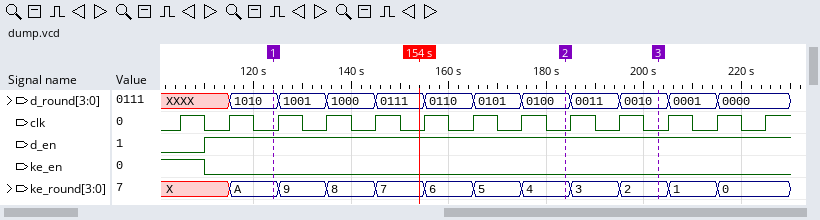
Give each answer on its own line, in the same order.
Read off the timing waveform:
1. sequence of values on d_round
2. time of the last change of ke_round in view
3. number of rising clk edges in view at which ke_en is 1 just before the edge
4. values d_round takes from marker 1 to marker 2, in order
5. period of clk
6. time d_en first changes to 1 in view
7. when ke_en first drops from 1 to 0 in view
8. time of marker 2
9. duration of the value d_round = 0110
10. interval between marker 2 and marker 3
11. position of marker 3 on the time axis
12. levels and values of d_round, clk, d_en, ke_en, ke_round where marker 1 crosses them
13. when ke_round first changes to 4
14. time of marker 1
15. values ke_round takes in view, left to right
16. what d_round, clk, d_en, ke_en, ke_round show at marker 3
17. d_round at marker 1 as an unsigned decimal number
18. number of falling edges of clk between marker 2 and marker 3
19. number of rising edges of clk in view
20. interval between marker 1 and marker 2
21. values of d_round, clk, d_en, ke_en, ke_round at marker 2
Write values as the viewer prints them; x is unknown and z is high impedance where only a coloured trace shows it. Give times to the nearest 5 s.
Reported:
XXXX, 1010, 1001, 1000, 0111, 0110, 0101, 0100, 0011, 0010, 0001, 0000
215 s
1
1010, 1001, 1000, 0111, 0110, 0101, 0100
10 s
110 s
110 s
185 s
10 s
20 s
205 s
d_round=1010, clk=0, d_en=1, ke_en=0, ke_round=A
175 s
125 s
X, A, 9, 8, 7, 6, 5, 4, 3, 2, 1, 0
d_round=0010, clk=0, d_en=1, ke_en=0, ke_round=2
10
2
13
60 s
d_round=0100, clk=0, d_en=1, ke_en=0, ke_round=4
